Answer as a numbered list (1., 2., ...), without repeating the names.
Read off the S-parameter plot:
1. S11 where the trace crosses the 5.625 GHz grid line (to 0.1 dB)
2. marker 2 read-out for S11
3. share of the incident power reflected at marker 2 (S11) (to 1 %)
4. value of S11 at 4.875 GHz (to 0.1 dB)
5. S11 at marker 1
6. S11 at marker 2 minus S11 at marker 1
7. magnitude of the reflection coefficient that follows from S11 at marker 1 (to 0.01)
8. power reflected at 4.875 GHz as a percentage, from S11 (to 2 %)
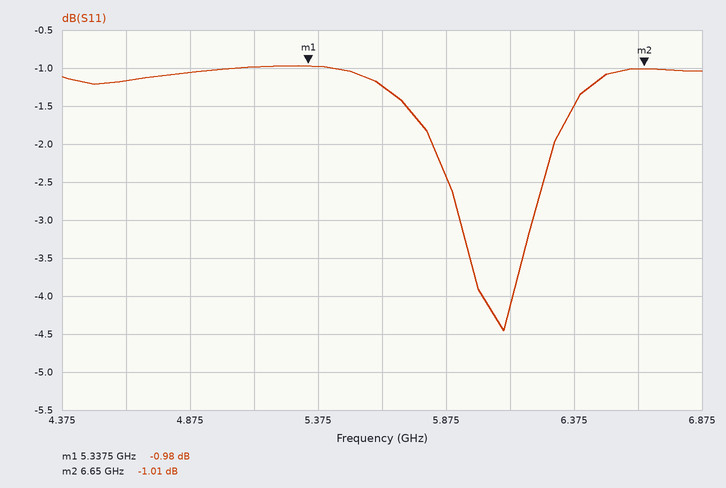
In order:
1. -1.2 dB
2. -1.01 dB
3. 79 %
4. -1.1 dB
5. -0.98 dB
6. -0.03 dB
7. 0.89
8. 78 %
